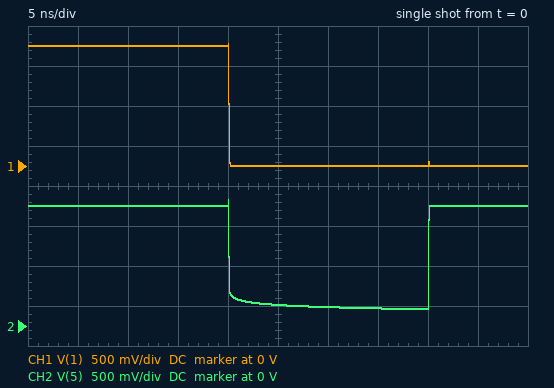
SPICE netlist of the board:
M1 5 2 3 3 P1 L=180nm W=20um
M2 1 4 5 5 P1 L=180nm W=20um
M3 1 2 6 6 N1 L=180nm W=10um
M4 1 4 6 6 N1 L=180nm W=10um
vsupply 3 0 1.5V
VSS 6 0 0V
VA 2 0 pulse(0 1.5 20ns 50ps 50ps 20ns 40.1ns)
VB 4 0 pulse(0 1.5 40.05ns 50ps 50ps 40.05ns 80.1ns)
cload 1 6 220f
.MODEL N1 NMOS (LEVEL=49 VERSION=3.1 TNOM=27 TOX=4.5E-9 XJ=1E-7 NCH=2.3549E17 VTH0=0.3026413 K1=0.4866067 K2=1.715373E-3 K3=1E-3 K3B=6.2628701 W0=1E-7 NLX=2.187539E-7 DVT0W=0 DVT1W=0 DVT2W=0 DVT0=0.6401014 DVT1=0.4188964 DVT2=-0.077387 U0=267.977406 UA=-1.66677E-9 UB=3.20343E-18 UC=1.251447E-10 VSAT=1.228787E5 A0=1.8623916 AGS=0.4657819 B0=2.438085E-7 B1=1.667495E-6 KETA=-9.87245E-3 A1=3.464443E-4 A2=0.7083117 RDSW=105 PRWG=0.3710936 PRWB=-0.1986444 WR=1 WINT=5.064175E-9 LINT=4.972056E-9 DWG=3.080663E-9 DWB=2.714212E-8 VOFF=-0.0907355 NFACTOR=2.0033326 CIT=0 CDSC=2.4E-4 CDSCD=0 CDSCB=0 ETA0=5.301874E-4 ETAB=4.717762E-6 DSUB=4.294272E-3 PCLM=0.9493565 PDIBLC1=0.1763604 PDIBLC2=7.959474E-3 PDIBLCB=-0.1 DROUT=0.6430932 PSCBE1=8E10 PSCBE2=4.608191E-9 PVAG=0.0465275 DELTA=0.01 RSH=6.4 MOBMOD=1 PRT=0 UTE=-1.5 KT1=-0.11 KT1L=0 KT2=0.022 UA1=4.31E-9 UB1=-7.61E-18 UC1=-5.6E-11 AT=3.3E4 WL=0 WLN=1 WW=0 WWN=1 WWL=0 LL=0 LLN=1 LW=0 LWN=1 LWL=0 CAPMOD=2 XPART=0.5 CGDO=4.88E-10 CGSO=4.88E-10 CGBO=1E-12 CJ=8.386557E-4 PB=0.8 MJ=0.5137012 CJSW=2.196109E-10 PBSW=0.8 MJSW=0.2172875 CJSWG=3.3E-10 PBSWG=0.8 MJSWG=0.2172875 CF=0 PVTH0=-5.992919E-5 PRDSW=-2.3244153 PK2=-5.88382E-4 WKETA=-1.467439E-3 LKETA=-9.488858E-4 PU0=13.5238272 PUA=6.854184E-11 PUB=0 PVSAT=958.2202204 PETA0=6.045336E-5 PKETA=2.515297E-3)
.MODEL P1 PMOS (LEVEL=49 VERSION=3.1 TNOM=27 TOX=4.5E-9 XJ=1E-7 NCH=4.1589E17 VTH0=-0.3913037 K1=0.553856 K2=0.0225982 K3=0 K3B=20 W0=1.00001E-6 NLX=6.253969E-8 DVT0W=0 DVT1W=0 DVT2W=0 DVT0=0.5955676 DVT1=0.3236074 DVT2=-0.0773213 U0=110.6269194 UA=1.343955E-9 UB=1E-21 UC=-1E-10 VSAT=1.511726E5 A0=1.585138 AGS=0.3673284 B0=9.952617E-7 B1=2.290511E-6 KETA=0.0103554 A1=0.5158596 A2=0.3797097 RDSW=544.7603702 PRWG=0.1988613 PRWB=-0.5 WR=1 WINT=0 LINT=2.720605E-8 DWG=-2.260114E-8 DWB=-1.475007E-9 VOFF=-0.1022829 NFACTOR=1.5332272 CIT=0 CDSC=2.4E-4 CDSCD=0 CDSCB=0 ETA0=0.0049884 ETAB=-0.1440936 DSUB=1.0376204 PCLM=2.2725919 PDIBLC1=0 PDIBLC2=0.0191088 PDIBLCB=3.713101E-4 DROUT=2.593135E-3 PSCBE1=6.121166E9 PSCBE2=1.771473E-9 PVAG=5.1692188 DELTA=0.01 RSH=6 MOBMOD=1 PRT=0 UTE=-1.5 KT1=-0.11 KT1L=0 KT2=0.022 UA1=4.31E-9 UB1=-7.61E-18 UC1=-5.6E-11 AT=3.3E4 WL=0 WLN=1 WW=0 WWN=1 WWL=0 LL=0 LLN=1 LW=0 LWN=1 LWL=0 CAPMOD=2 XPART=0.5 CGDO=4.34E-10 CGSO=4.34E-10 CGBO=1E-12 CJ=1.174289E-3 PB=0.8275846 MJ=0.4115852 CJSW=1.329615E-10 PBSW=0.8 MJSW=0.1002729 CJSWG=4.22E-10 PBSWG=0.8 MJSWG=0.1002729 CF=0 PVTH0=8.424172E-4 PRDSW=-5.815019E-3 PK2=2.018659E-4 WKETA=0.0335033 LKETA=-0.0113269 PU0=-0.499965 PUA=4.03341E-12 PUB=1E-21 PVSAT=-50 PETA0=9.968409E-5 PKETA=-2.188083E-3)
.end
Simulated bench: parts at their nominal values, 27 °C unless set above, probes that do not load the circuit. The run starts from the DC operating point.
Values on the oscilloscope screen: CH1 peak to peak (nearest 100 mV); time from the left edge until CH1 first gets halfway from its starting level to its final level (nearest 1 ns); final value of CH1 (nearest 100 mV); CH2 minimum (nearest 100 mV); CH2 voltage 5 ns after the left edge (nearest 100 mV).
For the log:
1.5 V
20 ns
0 V
200 mV
1.5 V
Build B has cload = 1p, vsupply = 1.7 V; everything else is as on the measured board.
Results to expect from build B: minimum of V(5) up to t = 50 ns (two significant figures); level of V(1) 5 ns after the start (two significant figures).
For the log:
230 mV
1.7 V
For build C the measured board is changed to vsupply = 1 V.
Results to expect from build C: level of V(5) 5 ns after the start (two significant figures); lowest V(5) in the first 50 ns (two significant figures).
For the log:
1.0 V
210 mV
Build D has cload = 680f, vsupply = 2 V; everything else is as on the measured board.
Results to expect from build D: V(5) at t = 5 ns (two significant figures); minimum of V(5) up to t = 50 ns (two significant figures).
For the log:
2.0 V
500 mV
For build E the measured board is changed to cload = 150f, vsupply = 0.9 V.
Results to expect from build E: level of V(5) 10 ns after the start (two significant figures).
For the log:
900 mV
